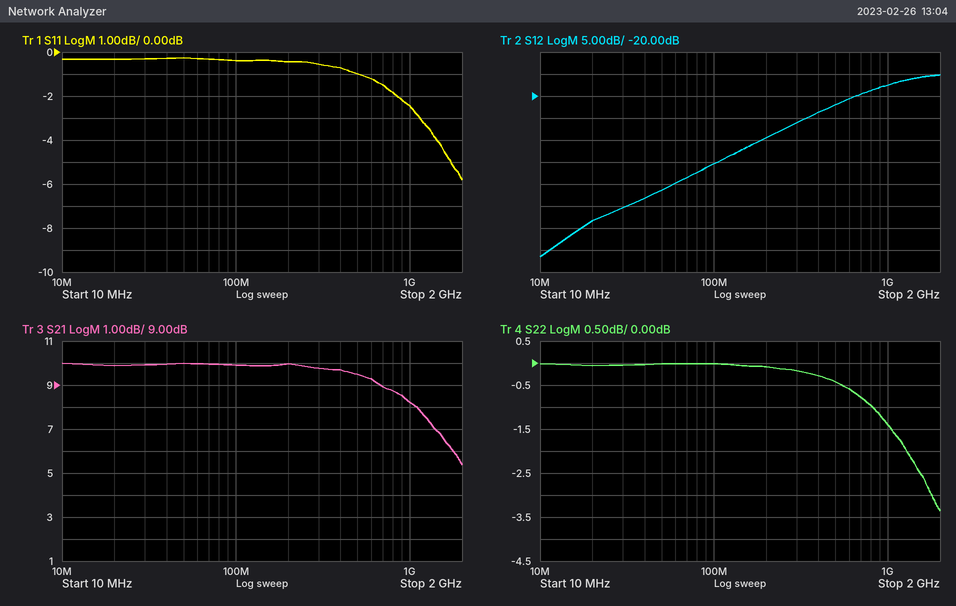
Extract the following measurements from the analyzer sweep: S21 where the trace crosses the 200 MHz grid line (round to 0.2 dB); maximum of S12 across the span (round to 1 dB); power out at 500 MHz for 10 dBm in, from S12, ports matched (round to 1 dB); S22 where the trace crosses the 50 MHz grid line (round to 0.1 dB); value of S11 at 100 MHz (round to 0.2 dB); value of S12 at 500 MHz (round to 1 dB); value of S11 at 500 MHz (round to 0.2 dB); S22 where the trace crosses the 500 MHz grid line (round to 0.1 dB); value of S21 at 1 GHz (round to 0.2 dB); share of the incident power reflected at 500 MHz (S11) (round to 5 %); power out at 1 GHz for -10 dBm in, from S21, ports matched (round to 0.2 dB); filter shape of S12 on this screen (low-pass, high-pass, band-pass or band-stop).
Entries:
10.0 dB
-15 dB
-12 dBm
0.0 dB
-0.4 dB
-22 dB
-1.0 dB
-0.4 dB
8.2 dB
80 %
-1.8 dBm
high-pass
